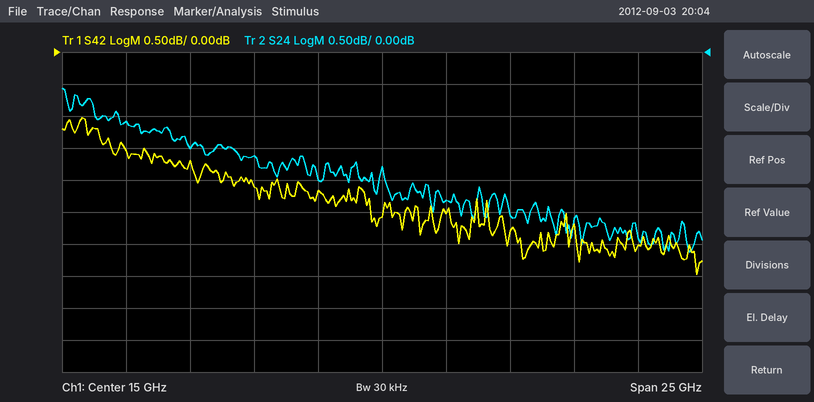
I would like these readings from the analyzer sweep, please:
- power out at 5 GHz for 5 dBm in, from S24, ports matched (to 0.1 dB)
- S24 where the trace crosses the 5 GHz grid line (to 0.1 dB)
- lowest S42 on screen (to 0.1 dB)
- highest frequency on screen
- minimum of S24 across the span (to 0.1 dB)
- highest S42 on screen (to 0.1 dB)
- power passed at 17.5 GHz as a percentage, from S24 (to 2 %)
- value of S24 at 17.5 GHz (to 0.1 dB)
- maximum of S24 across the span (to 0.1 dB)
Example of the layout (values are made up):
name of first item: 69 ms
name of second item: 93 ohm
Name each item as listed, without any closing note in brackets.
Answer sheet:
power out at 5 GHz for 5 dBm in, from S24, ports matched: 3.9 dBm
S24 where the trace crosses the 5 GHz grid line: -1.1 dB
lowest S42 on screen: -3.5 dB
highest frequency on screen: 27.5 GHz
minimum of S24 across the span: -3.1 dB
highest S42 on screen: -1.0 dB
power passed at 17.5 GHz as a percentage, from S24: 58 %
value of S24 at 17.5 GHz: -2.3 dB
maximum of S24 across the span: -0.6 dB
